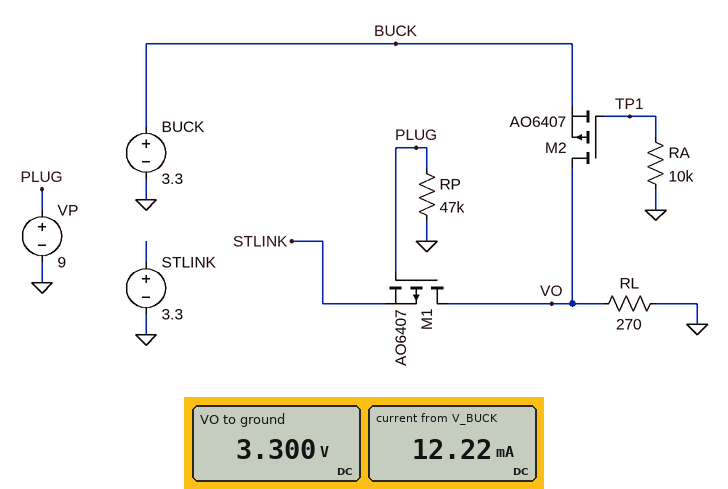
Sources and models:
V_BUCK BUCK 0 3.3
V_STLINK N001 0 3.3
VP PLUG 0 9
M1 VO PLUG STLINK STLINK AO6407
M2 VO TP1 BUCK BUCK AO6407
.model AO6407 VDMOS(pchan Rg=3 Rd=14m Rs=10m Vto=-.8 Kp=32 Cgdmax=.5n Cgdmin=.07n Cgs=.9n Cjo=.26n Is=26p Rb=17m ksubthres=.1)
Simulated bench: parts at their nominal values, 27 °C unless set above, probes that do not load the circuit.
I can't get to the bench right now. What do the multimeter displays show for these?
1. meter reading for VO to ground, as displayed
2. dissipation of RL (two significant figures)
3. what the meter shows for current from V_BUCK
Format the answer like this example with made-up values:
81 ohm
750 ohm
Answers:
3.300 V
40 mW
12.22 mA
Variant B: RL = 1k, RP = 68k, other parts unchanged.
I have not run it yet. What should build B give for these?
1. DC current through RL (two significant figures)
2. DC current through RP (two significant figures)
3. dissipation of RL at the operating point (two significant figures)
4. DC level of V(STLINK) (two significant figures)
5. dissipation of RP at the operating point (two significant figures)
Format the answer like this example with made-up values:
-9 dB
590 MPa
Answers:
3.3 mA
130 µA
11 mW
3.3 V
1.2 mW
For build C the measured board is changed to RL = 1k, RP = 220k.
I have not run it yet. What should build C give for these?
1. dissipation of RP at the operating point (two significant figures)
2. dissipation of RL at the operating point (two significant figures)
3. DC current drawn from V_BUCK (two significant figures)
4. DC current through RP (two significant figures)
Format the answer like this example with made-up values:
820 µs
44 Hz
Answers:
370 µW
11 mW
3.3 mA
41 µA
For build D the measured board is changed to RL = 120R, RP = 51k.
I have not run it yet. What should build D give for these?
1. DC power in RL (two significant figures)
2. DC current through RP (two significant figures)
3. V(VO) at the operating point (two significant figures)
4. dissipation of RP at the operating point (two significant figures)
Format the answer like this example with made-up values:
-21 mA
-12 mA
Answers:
91 mW
180 µA
3.3 V
1.6 mW
